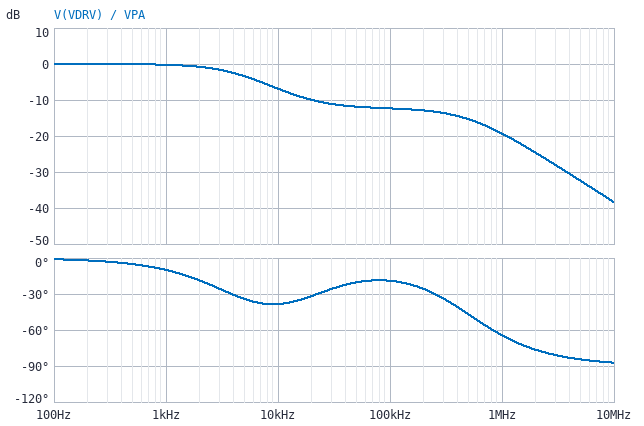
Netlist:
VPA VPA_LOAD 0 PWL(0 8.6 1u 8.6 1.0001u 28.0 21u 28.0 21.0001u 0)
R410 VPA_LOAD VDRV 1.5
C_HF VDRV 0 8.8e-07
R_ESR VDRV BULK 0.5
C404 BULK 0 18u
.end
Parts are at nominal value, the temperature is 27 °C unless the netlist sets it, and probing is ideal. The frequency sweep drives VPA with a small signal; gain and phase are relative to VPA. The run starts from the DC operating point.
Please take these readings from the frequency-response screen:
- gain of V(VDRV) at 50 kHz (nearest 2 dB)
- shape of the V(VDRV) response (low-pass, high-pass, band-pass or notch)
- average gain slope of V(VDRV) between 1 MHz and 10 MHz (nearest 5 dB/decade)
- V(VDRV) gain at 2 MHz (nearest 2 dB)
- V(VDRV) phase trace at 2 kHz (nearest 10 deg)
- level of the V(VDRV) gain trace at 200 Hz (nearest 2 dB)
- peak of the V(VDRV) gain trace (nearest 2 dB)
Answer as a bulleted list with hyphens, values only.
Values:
- -12 dB
- low-pass
- -20 dB/decade
- -24 dB
- -20 deg
- 0 dB
- 0 dB
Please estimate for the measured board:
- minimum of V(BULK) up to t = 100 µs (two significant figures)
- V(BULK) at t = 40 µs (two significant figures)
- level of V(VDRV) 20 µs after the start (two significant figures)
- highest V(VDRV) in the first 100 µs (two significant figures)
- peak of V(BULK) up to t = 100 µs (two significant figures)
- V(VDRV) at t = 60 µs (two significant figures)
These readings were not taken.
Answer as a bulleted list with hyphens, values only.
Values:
- 2.0 V
- 10 V
- 19 V
- 19 V
- 17 V
- 4.4 V
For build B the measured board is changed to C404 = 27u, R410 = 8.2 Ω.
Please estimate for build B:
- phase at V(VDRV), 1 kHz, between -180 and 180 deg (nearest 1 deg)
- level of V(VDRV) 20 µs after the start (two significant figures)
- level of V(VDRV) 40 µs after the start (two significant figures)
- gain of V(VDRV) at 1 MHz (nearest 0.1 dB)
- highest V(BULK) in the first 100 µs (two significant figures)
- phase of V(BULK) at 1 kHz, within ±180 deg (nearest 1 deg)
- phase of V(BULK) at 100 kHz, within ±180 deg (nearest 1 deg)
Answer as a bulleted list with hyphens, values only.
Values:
- -52 deg
- 11 V
- 8.9 V
- -33.8 dB
- 10 V
- -57 deg
- -104 deg
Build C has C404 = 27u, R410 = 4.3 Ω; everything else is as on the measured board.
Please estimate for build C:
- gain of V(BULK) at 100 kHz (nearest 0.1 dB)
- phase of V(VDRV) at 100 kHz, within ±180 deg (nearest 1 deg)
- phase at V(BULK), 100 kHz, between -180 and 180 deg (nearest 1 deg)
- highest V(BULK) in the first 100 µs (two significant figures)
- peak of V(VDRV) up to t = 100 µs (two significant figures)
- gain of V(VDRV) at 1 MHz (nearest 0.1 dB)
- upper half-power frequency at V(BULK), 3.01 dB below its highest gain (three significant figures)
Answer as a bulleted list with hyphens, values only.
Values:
- -38.7 dB
- -20 deg
- -103 deg
- 11 V
- 13 V
- -28.2 dB
- 1.20 kHz
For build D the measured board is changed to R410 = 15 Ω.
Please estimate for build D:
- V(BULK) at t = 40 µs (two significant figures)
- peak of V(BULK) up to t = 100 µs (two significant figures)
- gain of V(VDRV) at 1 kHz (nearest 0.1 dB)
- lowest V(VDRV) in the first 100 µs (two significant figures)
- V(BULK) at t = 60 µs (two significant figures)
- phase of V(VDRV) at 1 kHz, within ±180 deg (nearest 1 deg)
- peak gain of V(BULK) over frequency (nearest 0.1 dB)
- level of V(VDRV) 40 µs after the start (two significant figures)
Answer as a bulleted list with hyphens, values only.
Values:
- 9.3 V
- 9.9 V
- -6.4 dB
- 7.3 V
- 8.7 V
- -58 deg
- 0 dB
- 9.0 V
